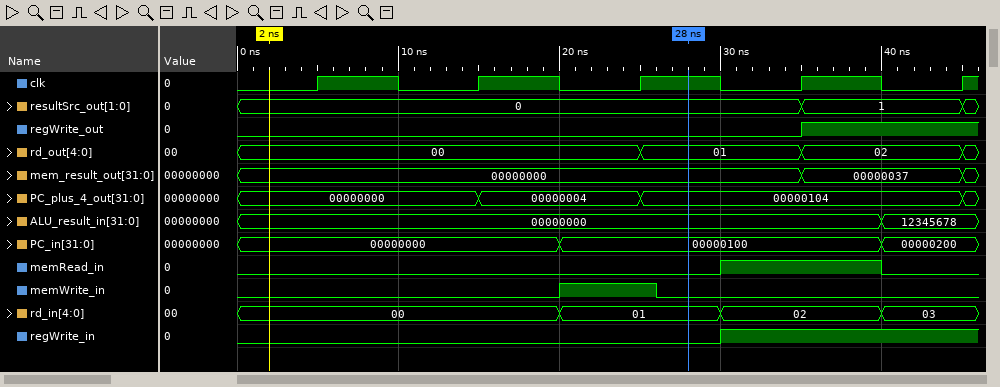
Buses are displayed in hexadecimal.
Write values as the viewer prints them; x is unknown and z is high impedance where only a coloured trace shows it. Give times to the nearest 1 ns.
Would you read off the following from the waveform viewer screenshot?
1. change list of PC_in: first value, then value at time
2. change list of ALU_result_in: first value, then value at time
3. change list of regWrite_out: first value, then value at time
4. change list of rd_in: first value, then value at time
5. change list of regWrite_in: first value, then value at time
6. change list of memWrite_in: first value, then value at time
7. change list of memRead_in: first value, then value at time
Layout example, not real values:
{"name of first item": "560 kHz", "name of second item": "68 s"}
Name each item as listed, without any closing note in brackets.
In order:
{"change list of PC_in: first value, then value at time": "00000000, 00000100 at 20 ns, 00000200 at 40 ns", "change list of ALU_result_in: first value, then value at time": "00000000, 12345678 at 40 ns", "change list of regWrite_out: first value, then value at time": "0, 1 at 35 ns", "change list of rd_in: first value, then value at time": "00, 01 at 20 ns, 02 at 30 ns, 03 at 40 ns", "change list of regWrite_in: first value, then value at time": "0, 1 at 30 ns", "change list of memWrite_in: first value, then value at time": "0, 1 at 20 ns, 0 at 26 ns", "change list of memRead_in: first value, then value at time": "0, 1 at 30 ns, 0 at 40 ns"}
